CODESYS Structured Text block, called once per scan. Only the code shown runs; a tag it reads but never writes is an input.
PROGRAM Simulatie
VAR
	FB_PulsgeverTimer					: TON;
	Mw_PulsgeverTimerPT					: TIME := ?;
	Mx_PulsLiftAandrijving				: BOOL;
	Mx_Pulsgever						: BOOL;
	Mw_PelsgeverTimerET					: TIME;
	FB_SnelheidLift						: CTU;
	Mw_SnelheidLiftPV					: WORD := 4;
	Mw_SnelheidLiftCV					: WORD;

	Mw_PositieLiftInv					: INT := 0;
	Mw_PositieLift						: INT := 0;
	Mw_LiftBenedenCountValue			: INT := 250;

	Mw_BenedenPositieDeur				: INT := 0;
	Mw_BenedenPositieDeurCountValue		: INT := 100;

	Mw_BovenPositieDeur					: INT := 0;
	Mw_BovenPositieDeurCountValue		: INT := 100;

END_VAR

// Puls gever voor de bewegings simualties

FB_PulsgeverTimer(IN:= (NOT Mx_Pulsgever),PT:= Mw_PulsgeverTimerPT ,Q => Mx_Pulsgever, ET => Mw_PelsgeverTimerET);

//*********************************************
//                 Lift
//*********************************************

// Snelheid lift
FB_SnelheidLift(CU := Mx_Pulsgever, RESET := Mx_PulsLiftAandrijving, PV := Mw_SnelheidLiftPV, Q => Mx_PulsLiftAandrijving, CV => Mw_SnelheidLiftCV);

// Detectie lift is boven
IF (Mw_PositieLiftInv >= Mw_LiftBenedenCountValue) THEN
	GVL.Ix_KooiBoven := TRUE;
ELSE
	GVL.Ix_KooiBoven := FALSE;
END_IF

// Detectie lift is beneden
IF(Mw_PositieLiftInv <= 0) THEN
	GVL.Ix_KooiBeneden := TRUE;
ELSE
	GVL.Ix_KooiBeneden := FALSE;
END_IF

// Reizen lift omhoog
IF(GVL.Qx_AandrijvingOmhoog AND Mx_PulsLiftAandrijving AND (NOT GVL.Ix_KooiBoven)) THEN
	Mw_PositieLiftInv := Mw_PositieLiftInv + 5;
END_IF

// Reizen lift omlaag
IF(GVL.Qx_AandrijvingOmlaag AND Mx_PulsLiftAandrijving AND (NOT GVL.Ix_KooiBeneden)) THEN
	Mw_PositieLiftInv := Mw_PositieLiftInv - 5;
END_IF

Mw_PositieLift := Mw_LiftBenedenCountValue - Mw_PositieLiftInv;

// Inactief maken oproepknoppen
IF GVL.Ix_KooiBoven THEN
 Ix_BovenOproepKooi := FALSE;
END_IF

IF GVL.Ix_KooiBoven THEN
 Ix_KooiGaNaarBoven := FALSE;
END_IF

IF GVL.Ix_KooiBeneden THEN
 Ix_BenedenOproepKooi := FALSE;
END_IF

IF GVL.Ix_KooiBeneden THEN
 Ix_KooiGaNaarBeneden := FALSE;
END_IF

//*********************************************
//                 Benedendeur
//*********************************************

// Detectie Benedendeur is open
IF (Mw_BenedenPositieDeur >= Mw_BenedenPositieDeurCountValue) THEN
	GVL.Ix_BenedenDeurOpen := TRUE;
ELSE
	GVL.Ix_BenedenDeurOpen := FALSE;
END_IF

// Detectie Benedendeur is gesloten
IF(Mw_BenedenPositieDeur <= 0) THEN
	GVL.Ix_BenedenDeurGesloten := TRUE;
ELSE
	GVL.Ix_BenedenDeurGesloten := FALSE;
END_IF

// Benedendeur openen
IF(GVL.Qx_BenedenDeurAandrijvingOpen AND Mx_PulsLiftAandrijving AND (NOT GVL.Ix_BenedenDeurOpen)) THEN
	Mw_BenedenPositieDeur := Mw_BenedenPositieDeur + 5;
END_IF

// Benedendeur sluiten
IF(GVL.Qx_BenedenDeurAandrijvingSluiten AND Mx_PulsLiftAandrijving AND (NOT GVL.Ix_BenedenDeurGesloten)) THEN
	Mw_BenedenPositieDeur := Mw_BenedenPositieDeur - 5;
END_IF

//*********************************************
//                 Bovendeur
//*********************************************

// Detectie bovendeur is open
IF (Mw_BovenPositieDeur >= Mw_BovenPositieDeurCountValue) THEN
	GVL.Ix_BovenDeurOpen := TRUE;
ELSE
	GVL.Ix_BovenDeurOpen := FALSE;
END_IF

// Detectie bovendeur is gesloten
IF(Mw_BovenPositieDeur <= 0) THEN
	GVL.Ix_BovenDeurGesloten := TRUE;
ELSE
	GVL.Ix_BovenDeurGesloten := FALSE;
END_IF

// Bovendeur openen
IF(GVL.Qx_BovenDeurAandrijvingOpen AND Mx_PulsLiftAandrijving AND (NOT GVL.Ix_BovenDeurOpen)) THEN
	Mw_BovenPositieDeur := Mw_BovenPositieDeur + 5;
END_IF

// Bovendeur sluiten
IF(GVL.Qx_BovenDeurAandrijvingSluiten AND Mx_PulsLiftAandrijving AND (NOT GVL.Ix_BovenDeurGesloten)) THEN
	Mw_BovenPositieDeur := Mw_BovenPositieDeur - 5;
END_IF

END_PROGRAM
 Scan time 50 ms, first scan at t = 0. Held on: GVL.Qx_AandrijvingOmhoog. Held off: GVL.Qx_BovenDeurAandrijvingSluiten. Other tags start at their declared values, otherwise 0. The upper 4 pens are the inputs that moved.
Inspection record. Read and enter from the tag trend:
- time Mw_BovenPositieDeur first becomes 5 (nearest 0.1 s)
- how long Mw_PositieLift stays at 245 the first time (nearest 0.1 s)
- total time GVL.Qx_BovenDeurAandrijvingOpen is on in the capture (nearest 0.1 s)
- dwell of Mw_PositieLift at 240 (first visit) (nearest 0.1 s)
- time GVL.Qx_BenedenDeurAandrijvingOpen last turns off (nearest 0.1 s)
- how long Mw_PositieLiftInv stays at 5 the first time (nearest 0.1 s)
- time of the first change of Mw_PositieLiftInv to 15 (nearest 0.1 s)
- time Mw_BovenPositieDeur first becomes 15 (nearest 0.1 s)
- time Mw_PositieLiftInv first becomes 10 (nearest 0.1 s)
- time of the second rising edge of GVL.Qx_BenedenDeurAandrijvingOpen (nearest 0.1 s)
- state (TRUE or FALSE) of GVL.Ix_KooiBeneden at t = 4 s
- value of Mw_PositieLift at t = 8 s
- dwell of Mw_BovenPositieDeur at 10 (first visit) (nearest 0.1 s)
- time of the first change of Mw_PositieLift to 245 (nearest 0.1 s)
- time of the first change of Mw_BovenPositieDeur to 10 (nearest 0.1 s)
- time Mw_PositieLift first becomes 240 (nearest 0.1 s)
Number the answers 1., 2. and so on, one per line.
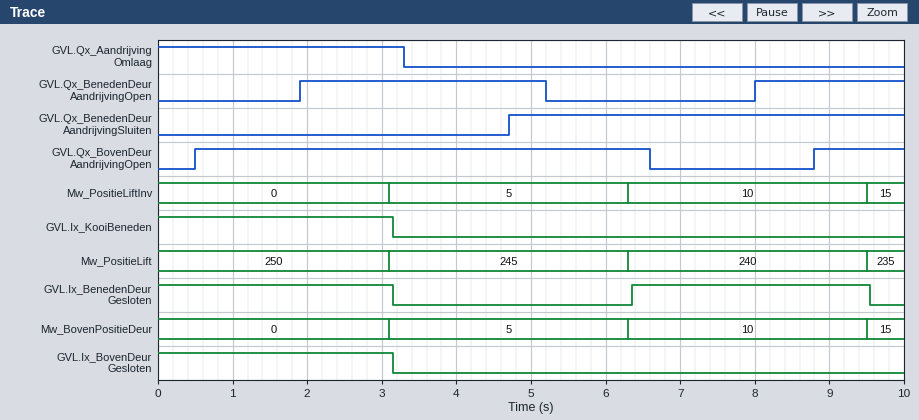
1. 3.1 s
2. 3.2 s
3. 7.3 s
4. 3.2 s
5. 5.2 s
6. 3.2 s
7. 9.5 s
8. 9.5 s
9. 6.3 s
10. 8.0 s
11. FALSE
12. 240
13. 3.2 s
14. 3.1 s
15. 6.3 s
16. 6.3 s
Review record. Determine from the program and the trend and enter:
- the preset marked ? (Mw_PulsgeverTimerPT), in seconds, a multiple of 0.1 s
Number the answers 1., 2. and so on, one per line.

1. 0.7 s
